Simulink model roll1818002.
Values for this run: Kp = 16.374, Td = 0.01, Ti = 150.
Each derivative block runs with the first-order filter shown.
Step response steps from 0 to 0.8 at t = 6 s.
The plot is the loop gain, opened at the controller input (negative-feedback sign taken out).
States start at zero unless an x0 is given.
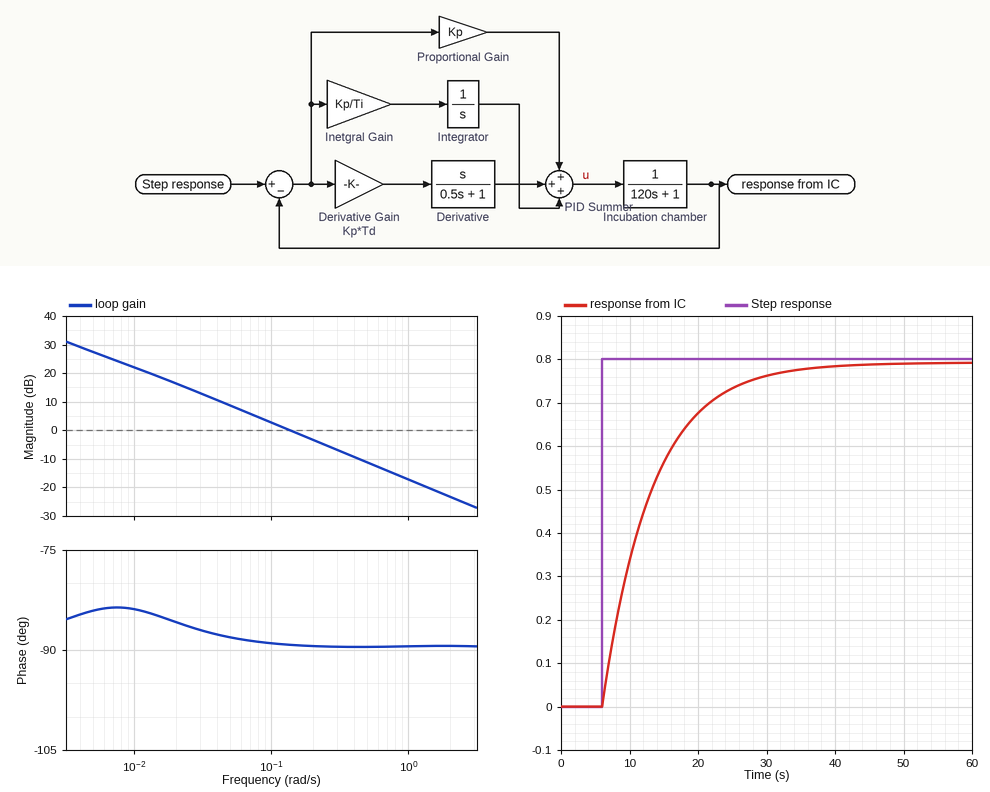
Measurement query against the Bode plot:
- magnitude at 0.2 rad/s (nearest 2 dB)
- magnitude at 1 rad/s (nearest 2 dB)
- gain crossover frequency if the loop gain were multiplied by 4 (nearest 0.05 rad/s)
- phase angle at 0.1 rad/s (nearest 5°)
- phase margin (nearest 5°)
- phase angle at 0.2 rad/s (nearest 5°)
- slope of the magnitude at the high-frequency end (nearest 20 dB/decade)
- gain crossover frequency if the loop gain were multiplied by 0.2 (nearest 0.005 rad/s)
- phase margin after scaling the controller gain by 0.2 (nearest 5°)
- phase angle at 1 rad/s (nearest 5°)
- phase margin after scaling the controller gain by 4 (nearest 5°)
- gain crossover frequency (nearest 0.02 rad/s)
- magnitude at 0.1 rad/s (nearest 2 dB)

-4 dB
-18 dB
0.55 rad/s
-90°
90°
-90°
-20 dB/decade
0.025 rad/s
95°
-90°
90°
0.14 rad/s
2 dB
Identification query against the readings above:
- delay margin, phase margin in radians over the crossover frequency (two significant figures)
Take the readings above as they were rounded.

11 s
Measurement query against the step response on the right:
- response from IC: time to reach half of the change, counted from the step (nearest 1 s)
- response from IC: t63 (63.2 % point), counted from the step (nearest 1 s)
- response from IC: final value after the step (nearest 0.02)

5 s
7 s
0.80
